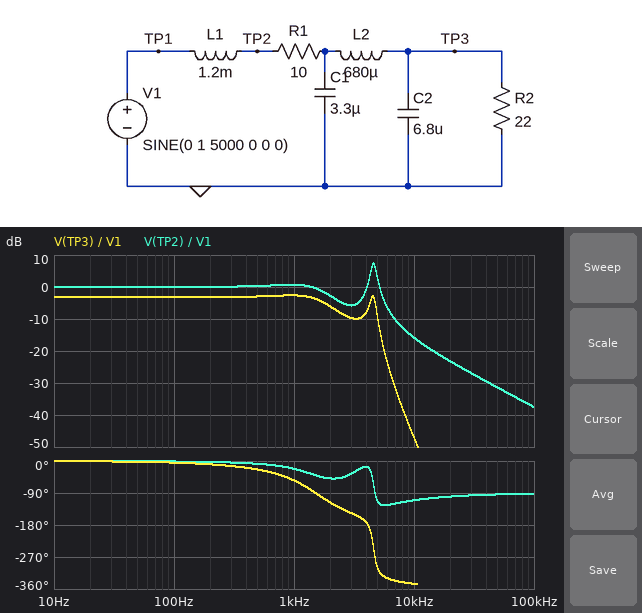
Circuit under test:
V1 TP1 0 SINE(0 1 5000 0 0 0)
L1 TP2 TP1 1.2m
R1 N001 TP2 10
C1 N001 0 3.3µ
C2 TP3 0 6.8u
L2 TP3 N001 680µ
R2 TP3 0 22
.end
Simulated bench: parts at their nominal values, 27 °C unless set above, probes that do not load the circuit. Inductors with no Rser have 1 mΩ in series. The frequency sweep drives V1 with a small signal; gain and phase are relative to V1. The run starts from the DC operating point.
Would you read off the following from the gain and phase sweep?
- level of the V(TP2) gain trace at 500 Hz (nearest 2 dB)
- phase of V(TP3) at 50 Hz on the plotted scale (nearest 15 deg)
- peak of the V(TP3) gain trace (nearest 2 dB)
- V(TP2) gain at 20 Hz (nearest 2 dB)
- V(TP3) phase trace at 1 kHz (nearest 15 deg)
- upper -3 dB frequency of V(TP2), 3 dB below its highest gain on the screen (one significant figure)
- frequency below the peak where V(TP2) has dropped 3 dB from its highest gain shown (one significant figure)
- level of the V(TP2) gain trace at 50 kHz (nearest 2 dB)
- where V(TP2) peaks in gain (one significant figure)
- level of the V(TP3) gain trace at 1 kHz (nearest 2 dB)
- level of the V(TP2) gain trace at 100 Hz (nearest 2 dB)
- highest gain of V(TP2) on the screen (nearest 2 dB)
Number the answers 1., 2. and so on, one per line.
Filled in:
1. 0 dB
2. 0 deg
3. -2 dB
4. 0 dB
5. -60 deg
6. 5 kHz
7. 4 kHz
8. -32 dB
9. 5 kHz
10. -2 dB
11. 0 dB
12. 8 dB
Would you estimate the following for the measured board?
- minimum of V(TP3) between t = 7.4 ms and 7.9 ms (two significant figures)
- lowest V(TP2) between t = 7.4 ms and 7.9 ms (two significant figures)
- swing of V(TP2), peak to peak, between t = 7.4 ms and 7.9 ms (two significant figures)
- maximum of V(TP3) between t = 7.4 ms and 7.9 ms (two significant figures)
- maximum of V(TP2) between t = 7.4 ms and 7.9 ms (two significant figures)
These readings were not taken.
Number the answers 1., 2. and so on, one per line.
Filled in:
1. -310 mV
2. -1.3 V
3. 2.6 V
4. 310 mV
5. 1.3 V
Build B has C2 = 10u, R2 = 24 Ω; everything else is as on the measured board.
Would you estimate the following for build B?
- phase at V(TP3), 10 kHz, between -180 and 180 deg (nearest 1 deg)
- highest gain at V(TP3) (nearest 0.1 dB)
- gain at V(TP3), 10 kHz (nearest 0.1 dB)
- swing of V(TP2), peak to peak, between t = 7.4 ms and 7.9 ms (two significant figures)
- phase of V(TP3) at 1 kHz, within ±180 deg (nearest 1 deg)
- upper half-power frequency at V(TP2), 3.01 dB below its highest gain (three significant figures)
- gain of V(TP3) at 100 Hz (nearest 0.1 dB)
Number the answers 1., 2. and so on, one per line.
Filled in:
1. 12 deg
2. -2.4 dB
3. -50.5 dB
4. 2.3 V
5. -67 deg
6. 4.68 kHz
7. -3.0 dB
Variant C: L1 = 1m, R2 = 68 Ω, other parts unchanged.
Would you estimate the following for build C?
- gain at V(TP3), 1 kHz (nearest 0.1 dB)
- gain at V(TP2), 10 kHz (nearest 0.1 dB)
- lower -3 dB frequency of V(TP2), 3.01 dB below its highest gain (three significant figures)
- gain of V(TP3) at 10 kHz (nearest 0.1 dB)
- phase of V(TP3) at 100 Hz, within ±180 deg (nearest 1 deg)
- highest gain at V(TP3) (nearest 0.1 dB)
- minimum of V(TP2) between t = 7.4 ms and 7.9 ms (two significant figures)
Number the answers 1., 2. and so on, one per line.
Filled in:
1. 0.5 dB
2. -14.2 dB
3. 4.47 kHz
4. -45.3 dB
5. -4 deg
6. 0.6 dB
7. -1.8 V
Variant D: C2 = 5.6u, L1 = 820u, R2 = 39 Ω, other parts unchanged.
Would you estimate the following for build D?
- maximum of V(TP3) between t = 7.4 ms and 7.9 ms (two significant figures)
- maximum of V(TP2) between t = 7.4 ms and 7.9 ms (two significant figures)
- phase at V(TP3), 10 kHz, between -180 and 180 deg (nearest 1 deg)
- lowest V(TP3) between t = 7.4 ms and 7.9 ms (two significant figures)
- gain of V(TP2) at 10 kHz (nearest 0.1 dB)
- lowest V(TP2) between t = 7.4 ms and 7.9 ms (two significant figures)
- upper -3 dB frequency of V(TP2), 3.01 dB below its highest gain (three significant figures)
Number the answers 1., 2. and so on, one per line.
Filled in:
1. 730 mV
2. 2.3 V
3. 17 deg
4. -730 mV
5. -12.3 dB
6. -2.3 V
7. 5.28 kHz
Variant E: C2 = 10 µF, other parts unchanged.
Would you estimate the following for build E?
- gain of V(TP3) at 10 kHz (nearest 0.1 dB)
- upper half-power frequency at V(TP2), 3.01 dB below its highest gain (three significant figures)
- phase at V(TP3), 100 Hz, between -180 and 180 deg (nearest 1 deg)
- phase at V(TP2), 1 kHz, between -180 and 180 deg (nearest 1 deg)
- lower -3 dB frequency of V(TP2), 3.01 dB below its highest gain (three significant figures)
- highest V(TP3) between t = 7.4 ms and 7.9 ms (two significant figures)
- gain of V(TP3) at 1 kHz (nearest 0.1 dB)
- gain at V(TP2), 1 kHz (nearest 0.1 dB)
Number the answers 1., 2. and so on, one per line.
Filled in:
1. -50.5 dB
2. 4.69 kHz
3. -5 deg
4. -26 deg
5. 4.24 kHz
6. 170 mV
7. -2.9 dB
8. 0.6 dB
